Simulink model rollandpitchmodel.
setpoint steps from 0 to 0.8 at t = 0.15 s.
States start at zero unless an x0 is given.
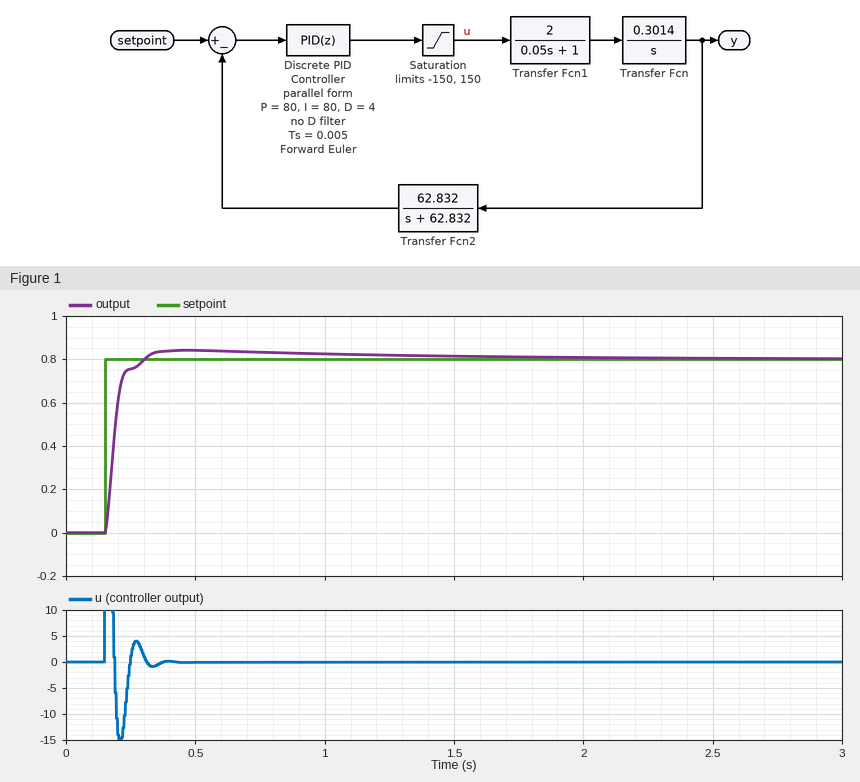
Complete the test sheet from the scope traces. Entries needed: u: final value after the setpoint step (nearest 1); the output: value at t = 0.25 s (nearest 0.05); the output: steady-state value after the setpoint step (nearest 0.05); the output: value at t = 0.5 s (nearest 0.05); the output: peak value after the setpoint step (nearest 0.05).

0
0.75
0.80
0.85
0.85
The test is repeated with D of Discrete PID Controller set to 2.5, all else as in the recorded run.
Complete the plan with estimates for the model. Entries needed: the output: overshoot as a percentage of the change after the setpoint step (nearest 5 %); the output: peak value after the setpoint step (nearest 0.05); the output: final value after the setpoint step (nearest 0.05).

20 %
0.95
0.80
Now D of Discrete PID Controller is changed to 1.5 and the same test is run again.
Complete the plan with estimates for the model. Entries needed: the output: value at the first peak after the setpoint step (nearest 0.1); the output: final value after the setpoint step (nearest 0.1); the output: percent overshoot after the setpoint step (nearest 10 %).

1.1
0.8
40 %
